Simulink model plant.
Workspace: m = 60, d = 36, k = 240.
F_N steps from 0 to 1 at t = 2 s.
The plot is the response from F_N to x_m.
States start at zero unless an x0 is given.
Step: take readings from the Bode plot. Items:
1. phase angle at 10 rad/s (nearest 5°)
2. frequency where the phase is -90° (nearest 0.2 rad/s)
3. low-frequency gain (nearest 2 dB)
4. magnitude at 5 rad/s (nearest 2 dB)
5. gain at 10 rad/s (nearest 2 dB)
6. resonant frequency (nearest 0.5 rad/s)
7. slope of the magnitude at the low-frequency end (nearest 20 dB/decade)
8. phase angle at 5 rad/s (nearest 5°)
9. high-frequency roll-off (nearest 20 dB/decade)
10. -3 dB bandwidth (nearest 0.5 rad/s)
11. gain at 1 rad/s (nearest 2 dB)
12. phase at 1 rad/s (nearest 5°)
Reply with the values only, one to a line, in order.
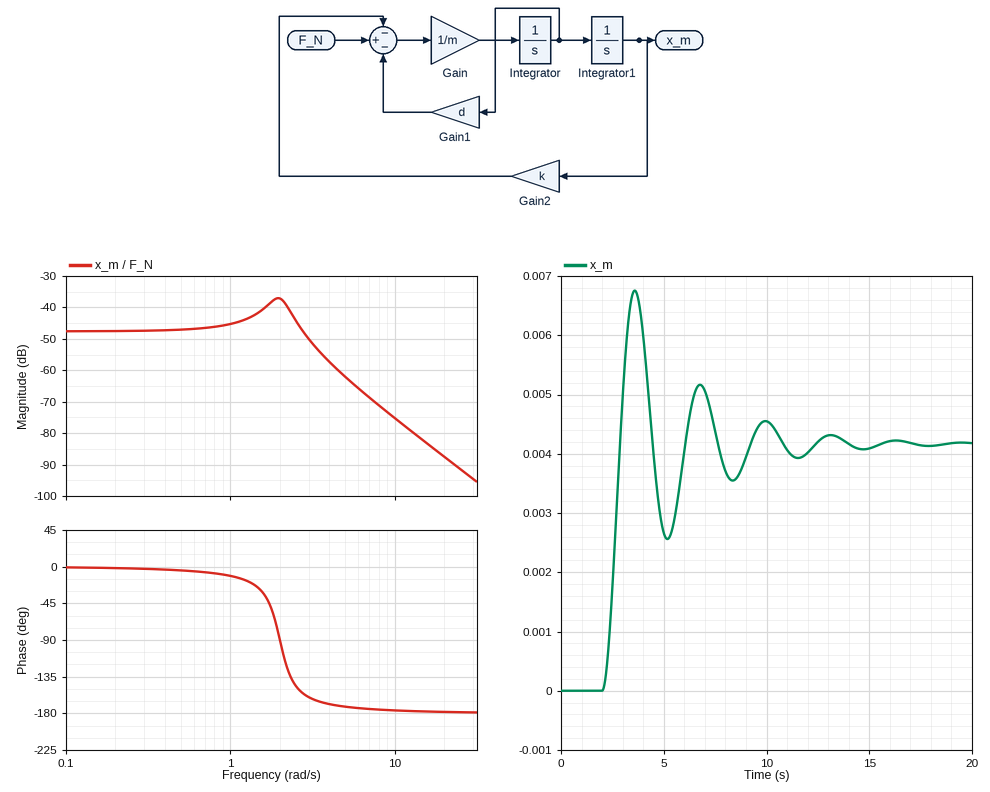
-175°
2.0 rad/s
-48 dB
-62 dB
-76 dB
2.0 rad/s
0 dB/decade
-170°
-40 dB/decade
3.0 rad/s
-46 dB
-10°
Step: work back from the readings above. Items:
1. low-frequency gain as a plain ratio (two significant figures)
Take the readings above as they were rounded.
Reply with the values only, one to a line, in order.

0.0040
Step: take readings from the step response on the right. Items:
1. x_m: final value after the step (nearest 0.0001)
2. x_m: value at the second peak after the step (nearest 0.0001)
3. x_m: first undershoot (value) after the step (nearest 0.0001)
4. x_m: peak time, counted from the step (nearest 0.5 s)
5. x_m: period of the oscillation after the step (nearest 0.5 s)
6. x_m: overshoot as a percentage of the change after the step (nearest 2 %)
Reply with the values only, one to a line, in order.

0.0042
0.0052
0.0026
1.5 s
3.0 s
62 %
